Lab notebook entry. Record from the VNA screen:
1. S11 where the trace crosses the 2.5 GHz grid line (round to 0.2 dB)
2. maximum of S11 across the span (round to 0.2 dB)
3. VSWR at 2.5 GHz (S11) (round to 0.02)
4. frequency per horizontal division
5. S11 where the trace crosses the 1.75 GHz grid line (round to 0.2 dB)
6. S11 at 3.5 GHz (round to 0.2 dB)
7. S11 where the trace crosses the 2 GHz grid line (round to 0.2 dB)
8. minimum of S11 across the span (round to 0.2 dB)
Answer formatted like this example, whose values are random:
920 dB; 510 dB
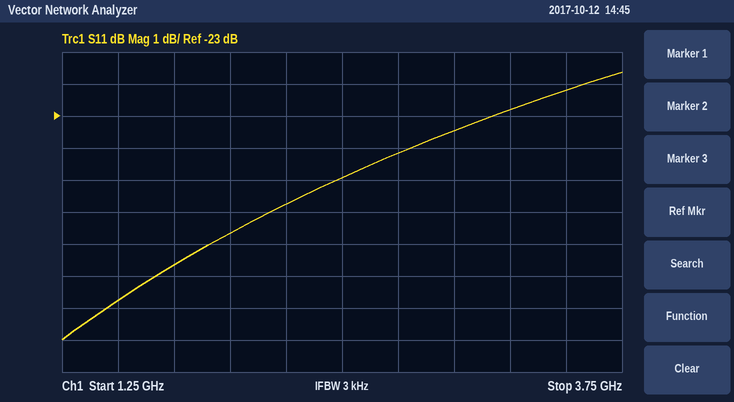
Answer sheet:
-25.0 dB; -21.6 dB; 1.12; 250 MHz; -27.6 dB; -22.2 dB; -26.6 dB; -30.0 dB
